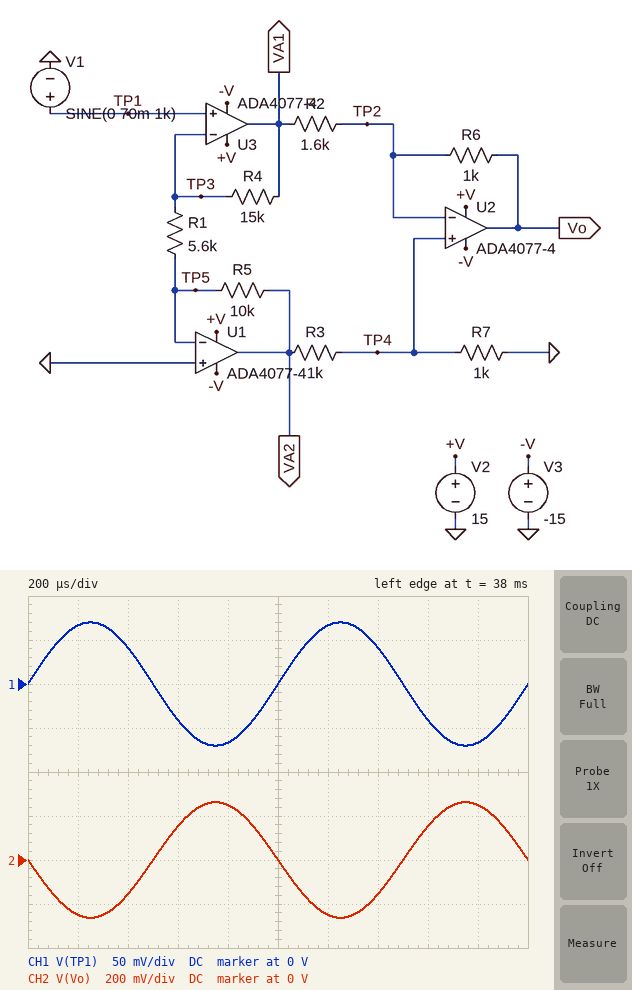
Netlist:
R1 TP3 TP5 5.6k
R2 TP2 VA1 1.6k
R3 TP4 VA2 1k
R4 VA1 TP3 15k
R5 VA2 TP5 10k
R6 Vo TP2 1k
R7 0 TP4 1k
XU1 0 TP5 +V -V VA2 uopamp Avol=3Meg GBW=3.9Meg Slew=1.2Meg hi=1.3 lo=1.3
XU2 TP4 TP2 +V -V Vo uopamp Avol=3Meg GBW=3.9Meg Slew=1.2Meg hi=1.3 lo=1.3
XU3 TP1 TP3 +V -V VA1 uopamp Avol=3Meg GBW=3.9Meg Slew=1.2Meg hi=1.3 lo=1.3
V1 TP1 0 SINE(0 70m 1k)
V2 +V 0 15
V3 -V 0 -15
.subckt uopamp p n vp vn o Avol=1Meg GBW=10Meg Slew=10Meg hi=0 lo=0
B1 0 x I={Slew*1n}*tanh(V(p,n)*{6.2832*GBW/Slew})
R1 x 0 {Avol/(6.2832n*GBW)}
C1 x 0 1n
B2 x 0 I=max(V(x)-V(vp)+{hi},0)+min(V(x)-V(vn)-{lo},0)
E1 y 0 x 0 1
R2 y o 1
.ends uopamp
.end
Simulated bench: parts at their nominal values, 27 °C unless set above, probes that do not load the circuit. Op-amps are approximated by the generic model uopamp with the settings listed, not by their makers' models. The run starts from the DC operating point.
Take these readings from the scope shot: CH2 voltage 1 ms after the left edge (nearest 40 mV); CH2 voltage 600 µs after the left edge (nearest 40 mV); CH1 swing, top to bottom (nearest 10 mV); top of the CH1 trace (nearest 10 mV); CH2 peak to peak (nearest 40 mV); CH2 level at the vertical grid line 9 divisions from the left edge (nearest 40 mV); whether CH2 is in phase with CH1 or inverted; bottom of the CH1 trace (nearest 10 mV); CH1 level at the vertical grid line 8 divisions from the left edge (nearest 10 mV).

0 V
160 mV
140 mV
70 mV
520 mV
240 mV
inverted
-70 mV
-40 mV
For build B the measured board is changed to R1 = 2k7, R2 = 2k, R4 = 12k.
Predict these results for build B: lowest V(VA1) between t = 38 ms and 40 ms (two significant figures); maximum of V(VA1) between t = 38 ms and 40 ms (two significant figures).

-380 mV
380 mV
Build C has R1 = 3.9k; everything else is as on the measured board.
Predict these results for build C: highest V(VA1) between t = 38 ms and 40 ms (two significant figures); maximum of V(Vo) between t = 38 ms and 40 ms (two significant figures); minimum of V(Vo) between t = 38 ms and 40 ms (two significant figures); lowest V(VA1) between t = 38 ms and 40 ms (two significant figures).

340 mV
360 mV
-360 mV
-340 mV
